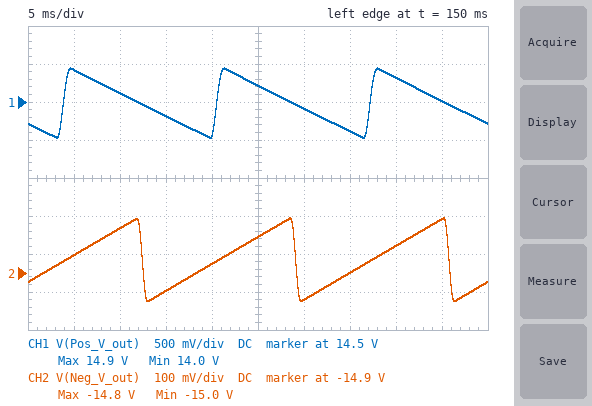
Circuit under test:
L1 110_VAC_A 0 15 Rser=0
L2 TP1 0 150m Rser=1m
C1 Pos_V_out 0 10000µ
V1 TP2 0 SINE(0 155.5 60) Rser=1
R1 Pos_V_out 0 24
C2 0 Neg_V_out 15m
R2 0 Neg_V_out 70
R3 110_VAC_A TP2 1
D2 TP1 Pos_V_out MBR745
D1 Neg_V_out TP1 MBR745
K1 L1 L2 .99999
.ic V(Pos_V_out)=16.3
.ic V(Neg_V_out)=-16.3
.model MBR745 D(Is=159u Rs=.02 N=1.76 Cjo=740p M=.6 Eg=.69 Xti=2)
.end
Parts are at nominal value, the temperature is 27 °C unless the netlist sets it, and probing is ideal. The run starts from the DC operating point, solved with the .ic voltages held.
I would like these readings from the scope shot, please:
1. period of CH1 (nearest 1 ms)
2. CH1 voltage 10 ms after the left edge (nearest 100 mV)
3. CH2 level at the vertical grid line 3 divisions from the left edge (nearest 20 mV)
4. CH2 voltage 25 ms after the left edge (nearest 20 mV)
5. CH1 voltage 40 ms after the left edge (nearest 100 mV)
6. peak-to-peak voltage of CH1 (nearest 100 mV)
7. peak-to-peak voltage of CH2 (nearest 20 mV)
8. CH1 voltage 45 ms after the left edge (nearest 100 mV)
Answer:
17 ms
14.6 V
-14.94 V
-14.80 V
14.8 V
900 mV
220 mV
14.5 V
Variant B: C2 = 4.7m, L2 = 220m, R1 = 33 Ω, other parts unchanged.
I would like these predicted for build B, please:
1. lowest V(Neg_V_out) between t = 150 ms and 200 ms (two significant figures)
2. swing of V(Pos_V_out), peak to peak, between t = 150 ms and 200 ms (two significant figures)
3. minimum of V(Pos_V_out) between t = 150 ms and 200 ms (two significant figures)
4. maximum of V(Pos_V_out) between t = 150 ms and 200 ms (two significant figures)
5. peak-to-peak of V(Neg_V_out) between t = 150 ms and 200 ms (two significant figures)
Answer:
-18 V
820 mV
17 V
18 V
840 mV
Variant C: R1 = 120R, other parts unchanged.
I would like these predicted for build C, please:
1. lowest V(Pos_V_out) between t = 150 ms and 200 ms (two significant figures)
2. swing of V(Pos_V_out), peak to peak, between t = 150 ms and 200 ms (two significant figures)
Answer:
15 V
190 mV
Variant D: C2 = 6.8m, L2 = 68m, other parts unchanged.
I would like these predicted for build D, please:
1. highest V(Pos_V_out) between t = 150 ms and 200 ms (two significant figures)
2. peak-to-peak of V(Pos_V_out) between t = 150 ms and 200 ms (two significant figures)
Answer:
10 V
610 mV
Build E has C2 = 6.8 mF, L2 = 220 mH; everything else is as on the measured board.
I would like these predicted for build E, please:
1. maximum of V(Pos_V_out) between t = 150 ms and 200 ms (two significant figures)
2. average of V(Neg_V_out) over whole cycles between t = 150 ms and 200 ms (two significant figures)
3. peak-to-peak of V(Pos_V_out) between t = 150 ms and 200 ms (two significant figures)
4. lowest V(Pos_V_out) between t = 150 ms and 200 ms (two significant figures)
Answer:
18 V
-18 V
1.1 V
17 V
